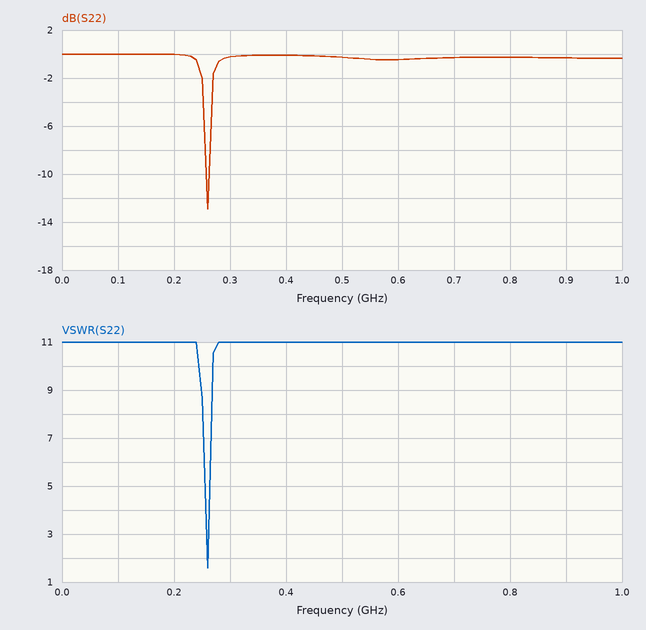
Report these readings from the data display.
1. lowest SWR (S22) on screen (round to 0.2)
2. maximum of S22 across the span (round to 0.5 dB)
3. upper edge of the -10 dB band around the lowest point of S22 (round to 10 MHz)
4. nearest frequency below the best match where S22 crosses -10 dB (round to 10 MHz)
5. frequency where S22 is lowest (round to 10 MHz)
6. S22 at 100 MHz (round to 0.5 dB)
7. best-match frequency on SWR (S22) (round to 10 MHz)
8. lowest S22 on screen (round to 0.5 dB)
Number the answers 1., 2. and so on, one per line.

1. 1.6
2. 0.0 dB
3. 260 MHz
4. 260 MHz
5. 260 MHz
6. 0.0 dB
7. 260 MHz
8. -13.0 dB
